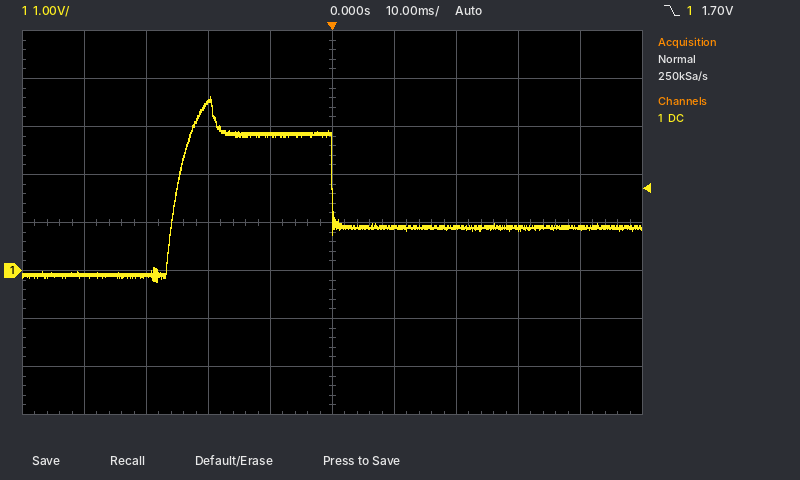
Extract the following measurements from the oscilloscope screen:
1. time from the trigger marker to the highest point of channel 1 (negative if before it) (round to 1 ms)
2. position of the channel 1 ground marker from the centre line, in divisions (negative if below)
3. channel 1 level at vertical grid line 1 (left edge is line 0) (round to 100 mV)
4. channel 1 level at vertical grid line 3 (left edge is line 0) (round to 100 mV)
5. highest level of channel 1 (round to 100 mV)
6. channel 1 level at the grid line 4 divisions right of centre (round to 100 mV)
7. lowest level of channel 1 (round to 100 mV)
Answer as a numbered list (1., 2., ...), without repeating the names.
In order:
1. -20 ms
2. -1.0 div
3. -100 mV
4. 3.5 V
5. 3.6 V
6. 900 mV
7. -200 mV
